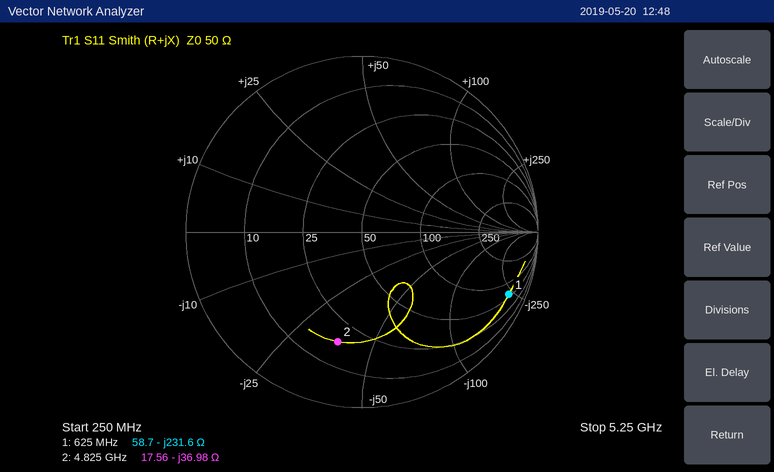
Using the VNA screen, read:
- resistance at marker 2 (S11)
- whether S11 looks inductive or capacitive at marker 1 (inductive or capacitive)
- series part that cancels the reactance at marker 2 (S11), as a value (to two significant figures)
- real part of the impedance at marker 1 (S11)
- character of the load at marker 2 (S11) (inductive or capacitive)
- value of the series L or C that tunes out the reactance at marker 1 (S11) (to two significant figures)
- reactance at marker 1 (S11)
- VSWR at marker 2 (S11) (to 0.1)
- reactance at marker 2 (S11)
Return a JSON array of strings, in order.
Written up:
["17.56 Ω", "capacitive", "1.2 nH", "58.7 Ω", "capacitive", "59 nH", "-231.6 Ω", "4.5", "-36.98 Ω"]
